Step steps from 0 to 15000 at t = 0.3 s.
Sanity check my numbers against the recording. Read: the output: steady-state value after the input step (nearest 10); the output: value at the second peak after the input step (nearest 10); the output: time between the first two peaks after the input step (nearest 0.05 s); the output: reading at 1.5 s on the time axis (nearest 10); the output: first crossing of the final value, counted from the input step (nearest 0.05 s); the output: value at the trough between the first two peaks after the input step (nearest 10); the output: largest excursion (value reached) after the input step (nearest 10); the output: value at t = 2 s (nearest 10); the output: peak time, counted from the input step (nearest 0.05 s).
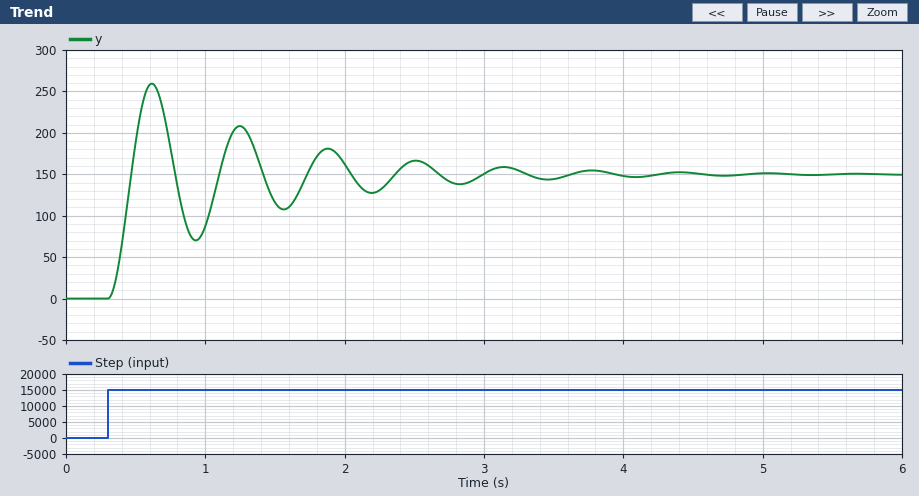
150
210
0.65 s
120
0.15 s
70
260
160
0.30 s
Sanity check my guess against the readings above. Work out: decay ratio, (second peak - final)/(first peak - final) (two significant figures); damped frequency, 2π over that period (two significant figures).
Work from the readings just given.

0.55
9.7 rad/s
